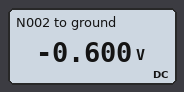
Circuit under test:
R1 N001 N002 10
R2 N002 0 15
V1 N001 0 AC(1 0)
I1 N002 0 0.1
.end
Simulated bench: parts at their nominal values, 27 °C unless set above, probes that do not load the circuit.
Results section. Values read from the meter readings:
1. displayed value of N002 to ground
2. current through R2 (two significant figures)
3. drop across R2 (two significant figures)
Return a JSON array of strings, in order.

["-0.600 V", "40 mA", "600 mV"]
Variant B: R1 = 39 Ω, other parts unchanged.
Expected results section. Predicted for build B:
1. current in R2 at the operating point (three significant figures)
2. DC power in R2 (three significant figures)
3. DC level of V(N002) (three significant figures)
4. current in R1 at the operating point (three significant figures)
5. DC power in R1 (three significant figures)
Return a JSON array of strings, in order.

["72.2 mA", "78.2 mW", "-1.08 V", "27.8 mA", "30.1 mW"]
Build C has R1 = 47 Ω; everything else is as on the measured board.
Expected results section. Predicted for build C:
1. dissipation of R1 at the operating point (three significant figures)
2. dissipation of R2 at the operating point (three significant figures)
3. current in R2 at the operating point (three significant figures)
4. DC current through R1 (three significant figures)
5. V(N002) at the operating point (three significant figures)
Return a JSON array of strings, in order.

["27.5 mW", "86.2 mW", "75.8 mA", "24.2 mA", "-1.14 V"]
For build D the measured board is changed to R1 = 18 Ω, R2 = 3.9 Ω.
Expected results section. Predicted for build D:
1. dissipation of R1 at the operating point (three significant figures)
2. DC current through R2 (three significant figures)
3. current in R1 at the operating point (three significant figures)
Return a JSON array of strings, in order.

["5.71 mW", "82.2 mA", "17.8 mA"]
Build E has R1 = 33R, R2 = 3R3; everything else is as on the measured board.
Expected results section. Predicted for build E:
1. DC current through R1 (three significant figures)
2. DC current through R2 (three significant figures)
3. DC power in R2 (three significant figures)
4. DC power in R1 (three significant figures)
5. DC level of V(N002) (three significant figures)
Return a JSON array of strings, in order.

["9.09 mA", "90.9 mA", "27.3 mW", "2.73 mW", "-300 mV"]
